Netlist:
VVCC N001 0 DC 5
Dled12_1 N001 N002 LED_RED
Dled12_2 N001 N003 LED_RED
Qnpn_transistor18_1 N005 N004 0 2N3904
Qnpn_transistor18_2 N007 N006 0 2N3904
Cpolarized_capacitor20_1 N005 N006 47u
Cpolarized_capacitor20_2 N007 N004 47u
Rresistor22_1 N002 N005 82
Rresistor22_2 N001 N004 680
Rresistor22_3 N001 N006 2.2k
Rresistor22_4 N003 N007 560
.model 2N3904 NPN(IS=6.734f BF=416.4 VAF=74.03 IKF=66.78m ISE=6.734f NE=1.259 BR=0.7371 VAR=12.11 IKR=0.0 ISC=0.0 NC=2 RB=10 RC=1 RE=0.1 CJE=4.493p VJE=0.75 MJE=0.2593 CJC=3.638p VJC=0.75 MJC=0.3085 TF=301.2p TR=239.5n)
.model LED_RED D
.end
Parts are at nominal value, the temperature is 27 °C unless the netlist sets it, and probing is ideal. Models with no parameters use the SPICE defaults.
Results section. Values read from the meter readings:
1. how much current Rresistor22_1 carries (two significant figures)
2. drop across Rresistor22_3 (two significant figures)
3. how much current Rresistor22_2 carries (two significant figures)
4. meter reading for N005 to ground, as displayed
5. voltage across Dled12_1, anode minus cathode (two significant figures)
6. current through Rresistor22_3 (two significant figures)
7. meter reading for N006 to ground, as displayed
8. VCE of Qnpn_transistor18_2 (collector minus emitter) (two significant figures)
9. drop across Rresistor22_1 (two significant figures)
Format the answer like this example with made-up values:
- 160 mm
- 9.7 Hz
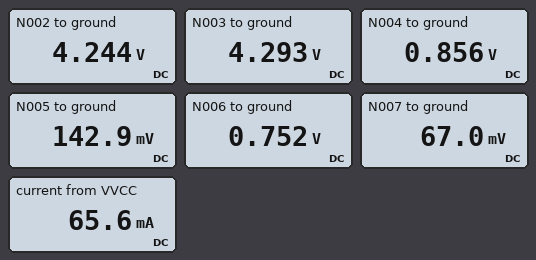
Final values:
- 50 mA
- 4.2 V
- 6.1 mA
- 142.9 mV
- 760 mV
- 1.9 mA
- 0.752 V
- 67 mV
- 4.1 V
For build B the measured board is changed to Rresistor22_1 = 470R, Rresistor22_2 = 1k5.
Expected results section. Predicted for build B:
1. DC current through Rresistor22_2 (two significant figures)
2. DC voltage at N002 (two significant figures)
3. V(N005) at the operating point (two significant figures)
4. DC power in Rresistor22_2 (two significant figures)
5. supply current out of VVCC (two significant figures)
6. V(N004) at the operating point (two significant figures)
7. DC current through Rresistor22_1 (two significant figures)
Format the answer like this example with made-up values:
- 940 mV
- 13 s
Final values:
- 2.8 mA
- 4.3 V
- 66 mV
- 12 mW
- 21 mA
- 770 mV
- 9.0 mA
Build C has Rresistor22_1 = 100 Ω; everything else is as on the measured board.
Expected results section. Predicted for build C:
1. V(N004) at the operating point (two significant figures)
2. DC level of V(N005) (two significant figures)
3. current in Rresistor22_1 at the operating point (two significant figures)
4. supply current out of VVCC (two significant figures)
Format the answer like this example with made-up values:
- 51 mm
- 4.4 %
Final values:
- 850 mV
- 130 mV
- 41 mA
- 57 mA
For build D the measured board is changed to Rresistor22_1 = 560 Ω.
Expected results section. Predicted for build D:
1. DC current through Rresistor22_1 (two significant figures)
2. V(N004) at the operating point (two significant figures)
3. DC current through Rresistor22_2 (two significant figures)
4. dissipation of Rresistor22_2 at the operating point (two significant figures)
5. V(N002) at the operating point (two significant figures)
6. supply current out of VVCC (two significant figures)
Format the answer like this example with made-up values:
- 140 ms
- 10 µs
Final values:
- 7.6 mA
- 810 mV
- 6.2 mA
- 26 mW
- 4.3 V
- 23 mA
